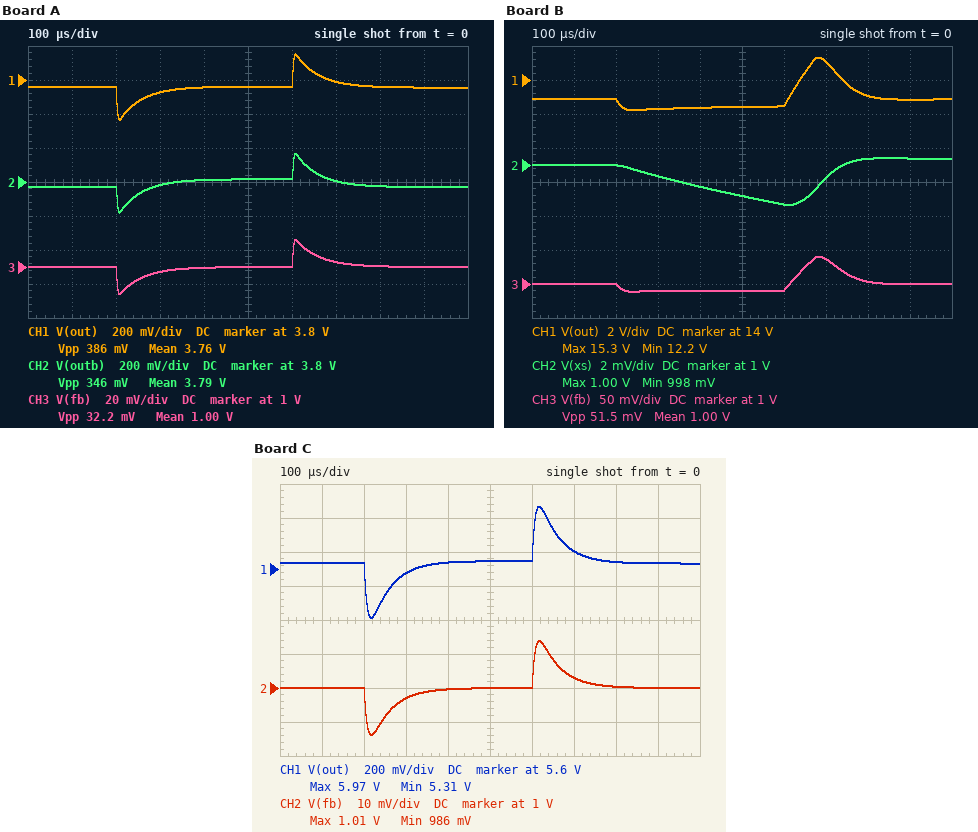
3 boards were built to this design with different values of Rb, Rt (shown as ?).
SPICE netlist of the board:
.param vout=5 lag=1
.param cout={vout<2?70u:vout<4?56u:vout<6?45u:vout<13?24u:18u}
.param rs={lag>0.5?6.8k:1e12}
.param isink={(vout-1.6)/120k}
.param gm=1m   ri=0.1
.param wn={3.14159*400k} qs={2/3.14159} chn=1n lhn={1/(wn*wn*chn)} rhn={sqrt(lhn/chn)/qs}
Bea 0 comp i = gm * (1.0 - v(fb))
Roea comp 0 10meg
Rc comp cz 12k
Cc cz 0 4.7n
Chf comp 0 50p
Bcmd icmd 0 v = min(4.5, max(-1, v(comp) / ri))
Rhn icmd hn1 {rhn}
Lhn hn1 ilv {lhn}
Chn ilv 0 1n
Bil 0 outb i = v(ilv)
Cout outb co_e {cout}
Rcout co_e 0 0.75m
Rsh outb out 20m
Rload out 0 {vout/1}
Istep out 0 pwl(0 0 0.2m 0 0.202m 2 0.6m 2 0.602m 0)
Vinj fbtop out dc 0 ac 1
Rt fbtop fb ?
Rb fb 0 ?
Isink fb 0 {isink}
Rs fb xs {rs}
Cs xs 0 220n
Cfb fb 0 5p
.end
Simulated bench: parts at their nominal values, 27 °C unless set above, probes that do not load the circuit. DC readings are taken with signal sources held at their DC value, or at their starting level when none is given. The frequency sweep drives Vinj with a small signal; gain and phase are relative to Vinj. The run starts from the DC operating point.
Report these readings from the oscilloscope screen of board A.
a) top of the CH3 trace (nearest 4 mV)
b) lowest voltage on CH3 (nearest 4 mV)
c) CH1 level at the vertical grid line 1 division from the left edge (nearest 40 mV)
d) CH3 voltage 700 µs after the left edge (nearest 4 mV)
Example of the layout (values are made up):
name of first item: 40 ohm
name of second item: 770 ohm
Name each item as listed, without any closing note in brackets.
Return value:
top of the CH3 trace: 1.016 V
lowest voltage on CH3: 984 mV
CH1 level at the vertical grid line 1 division from the left edge: 3.76 V
CH3 voltage 700 µs after the left edge: 1.004 V
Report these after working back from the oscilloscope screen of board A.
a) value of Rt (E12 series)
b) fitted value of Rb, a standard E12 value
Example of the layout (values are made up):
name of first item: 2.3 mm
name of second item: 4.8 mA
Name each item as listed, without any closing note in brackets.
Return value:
value of Rt: 68 kΩ
fitted value of Rb, a standard E12 value: 82 kΩ
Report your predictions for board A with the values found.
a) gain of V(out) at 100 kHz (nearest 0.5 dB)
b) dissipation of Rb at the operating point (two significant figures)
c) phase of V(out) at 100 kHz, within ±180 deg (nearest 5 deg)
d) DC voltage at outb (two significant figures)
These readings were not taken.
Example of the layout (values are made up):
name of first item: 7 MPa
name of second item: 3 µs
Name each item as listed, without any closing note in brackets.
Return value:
gain of V(out) at 100 kHz: -7.5 dB
dissipation of Rb at the operating point: 12 µW
phase of V(out) at 100 kHz, within ±180 deg: 30 deg
DC voltage at outb: 3.8 V
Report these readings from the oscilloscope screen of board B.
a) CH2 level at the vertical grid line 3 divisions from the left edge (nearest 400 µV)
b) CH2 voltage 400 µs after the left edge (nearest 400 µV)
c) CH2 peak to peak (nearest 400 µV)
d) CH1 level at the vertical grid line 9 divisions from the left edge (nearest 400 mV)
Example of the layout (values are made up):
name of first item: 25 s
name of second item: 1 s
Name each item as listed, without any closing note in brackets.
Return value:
CH2 level at the vertical grid line 3 divisions from the left edge: 999.2 mV
CH2 voltage 400 µs after the left edge: 998.8 mV
CH2 peak to peak: 2.8 mV
CH1 level at the vertical grid line 9 divisions from the left edge: 12.8 V
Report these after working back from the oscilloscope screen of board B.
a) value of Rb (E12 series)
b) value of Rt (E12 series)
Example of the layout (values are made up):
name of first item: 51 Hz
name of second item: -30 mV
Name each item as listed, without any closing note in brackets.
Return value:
value of Rb: 470 kΩ
value of Rt: 390 kΩ
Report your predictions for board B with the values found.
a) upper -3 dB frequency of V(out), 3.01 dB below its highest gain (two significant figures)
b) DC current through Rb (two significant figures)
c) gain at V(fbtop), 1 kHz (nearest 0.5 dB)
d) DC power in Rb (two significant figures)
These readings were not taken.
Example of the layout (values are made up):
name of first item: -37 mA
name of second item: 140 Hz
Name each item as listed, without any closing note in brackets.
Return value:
upper -3 dB frequency of V(out), 3.01 dB below its highest gain: 8.3 kHz
DC current through Rb: 2.1 µA
gain at V(fbtop), 1 kHz: -24.5 dB
DC power in Rb: 2.1 µW
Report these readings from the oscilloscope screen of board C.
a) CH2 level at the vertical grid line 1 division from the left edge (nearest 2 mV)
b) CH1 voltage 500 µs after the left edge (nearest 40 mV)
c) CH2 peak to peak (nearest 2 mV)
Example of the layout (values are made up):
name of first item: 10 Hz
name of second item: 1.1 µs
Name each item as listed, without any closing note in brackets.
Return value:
CH2 level at the vertical grid line 1 division from the left edge: 1.000 V
CH1 voltage 500 µs after the left edge: 5.64 V
CH2 peak to peak: 28 mV
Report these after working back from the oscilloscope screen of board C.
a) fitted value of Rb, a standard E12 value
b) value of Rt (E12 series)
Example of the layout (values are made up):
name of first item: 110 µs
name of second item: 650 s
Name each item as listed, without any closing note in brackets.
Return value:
fitted value of Rb, a standard E12 value: 390 kΩ
value of Rt: 150 kΩ
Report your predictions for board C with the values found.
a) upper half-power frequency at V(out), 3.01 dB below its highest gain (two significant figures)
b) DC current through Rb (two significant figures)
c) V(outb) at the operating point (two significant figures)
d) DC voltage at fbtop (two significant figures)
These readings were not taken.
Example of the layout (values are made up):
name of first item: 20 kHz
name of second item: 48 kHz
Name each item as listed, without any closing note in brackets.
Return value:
upper half-power frequency at V(out), 3.01 dB below its highest gain: 22 kHz
DC current through Rb: 2.6 µA
V(outb) at the operating point: 5.7 V
DC voltage at fbtop: 5.6 V
